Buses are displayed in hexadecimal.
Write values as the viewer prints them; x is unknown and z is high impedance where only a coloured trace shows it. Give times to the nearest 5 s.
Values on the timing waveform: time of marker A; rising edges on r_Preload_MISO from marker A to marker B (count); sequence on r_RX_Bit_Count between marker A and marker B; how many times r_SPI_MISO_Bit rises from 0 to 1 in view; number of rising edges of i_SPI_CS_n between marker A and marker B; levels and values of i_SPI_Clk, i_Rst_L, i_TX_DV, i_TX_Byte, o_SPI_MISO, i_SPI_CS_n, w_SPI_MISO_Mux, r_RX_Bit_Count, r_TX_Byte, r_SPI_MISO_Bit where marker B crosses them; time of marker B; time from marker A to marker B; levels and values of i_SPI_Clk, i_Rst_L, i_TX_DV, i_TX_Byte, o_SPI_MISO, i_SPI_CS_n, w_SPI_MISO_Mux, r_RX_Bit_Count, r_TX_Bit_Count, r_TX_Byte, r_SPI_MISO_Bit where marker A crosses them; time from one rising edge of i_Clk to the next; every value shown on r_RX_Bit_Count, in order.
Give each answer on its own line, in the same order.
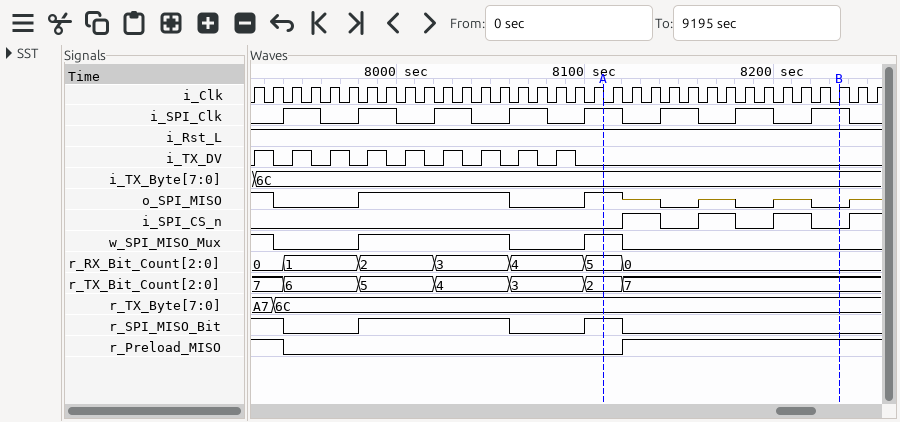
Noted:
8110 s
1
5, 0
2
3
i_SPI_Clk=1, i_Rst_L=1, i_TX_DV=0, i_TX_Byte=6C, o_SPI_MISO=0, i_SPI_CS_n=0, w_SPI_MISO_Mux=0, r_RX_Bit_Count=0, r_TX_Byte=6C, r_SPI_MISO_Bit=0
8235 s
125 s
i_SPI_Clk=1, i_Rst_L=1, i_TX_DV=0, i_TX_Byte=6C, o_SPI_MISO=1, i_SPI_CS_n=0, w_SPI_MISO_Mux=1, r_RX_Bit_Count=5, r_TX_Bit_Count=2, r_TX_Byte=6C, r_SPI_MISO_Bit=1
10 s
0, 1, 2, 3, 4, 5, 0
